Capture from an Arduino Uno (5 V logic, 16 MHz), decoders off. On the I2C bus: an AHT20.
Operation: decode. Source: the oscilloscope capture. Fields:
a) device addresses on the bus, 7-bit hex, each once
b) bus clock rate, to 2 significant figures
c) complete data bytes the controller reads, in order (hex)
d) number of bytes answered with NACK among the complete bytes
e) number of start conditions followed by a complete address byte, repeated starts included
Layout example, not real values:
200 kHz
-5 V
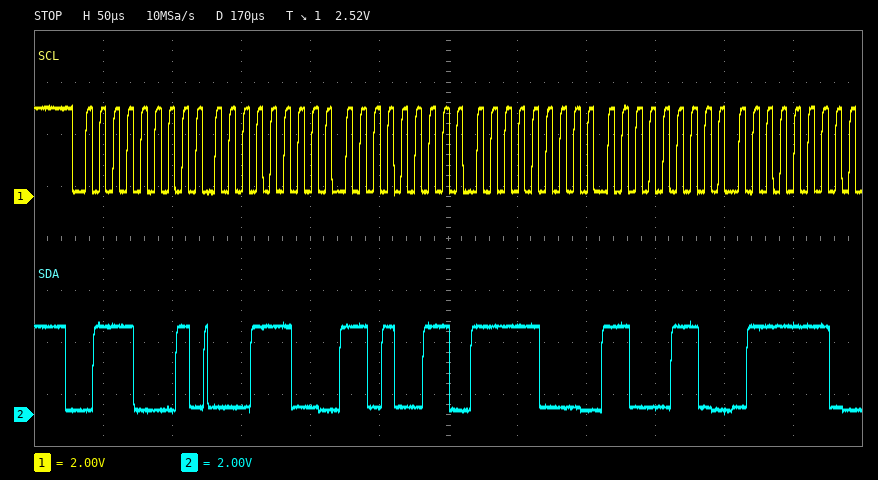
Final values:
0x38
100 kHz
1C D3 F8 C6 7E
0
1
